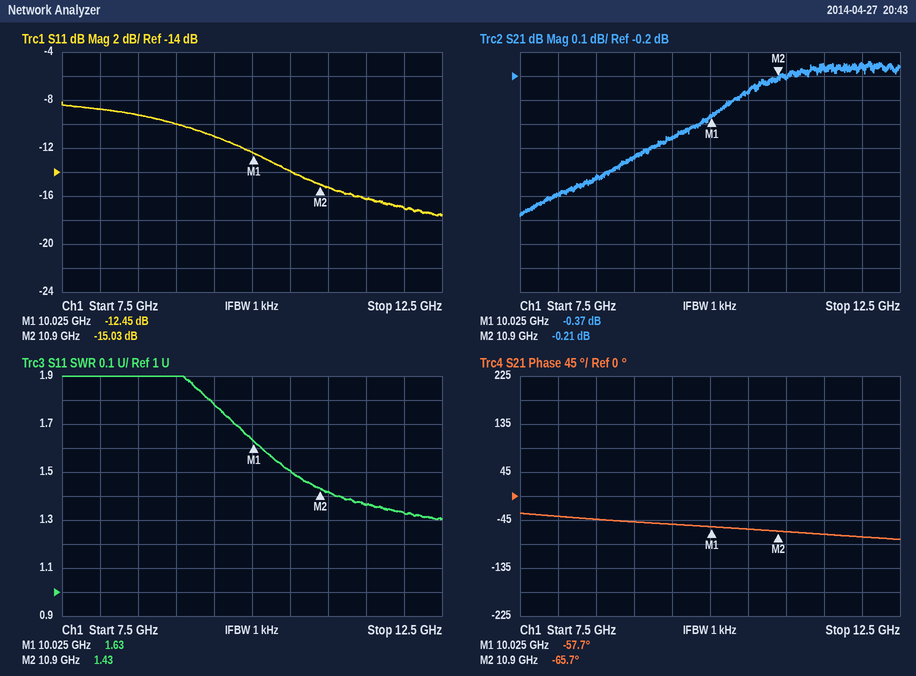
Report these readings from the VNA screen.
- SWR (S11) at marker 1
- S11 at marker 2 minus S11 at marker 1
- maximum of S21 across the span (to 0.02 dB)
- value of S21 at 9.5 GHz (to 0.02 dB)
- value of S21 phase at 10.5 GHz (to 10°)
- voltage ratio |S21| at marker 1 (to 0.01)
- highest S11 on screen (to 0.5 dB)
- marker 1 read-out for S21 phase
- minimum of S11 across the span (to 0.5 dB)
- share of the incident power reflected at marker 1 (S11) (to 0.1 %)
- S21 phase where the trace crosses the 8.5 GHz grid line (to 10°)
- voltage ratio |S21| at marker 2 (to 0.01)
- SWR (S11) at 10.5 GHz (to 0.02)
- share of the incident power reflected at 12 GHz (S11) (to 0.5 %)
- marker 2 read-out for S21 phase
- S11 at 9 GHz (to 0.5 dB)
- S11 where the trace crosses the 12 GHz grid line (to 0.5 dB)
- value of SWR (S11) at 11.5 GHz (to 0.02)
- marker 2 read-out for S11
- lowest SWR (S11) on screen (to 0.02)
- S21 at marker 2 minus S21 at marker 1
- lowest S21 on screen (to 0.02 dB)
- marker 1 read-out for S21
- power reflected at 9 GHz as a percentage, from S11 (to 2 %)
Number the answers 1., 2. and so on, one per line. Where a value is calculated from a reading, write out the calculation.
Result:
1. 1.63
2. -15.03 − (-12.45) = -2.58 dB
3. -0.14 dB
4. -0.46 dB
5. -60°
6. 10^(-0.37/20) ≈ 0.96
7. -8.0 dB
8. -57.7°
9. -17.5 dB
10. 10^(-12.45/10) ≈ 5.7 %
11. -40°
12. 10^(-0.21/20) ≈ 0.98
13. 1.50
14. 10^(-17/10) ≈ 2.0 %
15. -65.7°
16. -10.0 dB
17. -17.0 dB
18. 1.36
19. -15.03 dB
20. 1.30
21. -0.21 − (-0.37) = 0.16 dB
22. -0.78 dB
23. -0.37 dB
24. 10^(-10/10) ≈ 10 %
